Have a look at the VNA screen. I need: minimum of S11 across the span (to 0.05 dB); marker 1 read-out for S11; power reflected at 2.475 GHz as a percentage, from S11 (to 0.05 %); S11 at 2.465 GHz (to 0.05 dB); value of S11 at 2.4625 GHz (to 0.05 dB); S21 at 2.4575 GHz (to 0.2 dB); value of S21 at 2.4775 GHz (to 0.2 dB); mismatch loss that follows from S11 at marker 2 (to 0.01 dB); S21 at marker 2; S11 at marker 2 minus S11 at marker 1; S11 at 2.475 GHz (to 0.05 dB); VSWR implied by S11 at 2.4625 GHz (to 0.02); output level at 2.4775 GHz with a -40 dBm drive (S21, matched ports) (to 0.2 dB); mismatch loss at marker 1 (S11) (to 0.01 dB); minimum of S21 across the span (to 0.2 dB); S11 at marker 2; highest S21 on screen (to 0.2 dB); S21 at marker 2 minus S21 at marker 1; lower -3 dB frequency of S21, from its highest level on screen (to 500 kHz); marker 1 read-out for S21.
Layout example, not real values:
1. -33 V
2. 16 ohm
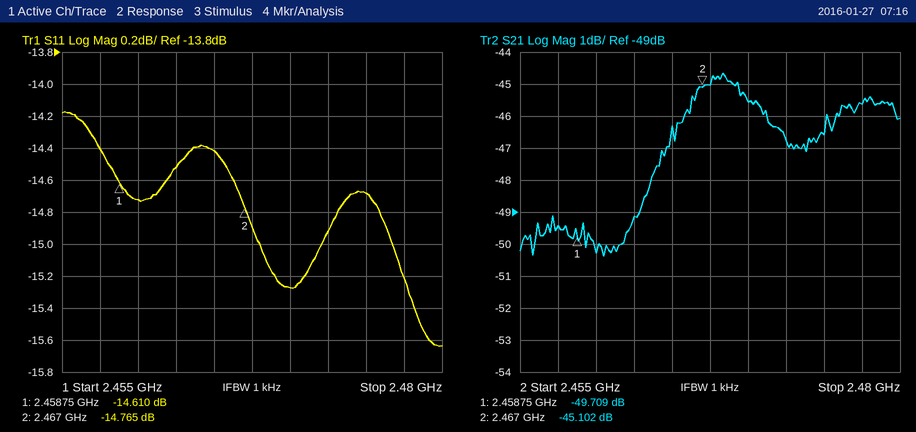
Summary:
1. -15.65 dB
2. -14.610 dB
3. 3.40 %
4. -14.40 dB
5. -14.50 dB
6. -49.4 dB
7. -45.6 dB
8. 0.15 dB
9. -45.102 dB
10. -0.155 dB
11. -14.70 dB
12. 1.46
13. -85.6 dBm
14. 0.15 dB
15. -50.4 dB
16. -14.765 dB
17. -44.6 dB
18. 4.607 dB
19. 2.4640 GHz
20. -49.709 dB
